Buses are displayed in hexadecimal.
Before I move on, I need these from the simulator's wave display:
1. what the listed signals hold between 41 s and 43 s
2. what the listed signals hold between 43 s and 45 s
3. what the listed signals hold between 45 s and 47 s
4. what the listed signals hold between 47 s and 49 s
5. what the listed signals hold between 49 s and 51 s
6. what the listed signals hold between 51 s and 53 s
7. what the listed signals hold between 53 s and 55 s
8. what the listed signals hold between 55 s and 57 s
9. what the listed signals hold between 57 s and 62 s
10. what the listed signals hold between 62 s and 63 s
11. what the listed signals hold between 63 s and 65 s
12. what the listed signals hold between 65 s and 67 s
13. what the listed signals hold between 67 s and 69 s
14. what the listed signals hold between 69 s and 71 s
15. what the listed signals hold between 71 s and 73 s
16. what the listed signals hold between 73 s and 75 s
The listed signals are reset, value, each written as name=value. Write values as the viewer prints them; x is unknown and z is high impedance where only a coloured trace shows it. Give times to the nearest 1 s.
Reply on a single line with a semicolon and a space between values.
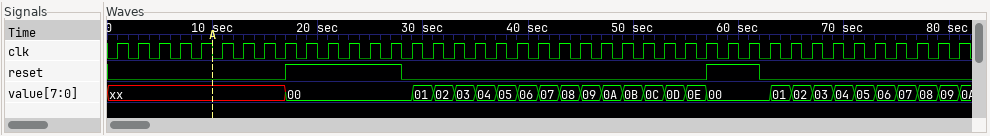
reset=0, value=07; reset=0, value=08; reset=0, value=09; reset=0, value=0A; reset=0, value=0B; reset=0, value=0C; reset=0, value=0D; reset=0, value=0E; reset=1, value=00; reset=0, value=00; reset=0, value=01; reset=0, value=02; reset=0, value=03; reset=0, value=04; reset=0, value=05; reset=0, value=06
